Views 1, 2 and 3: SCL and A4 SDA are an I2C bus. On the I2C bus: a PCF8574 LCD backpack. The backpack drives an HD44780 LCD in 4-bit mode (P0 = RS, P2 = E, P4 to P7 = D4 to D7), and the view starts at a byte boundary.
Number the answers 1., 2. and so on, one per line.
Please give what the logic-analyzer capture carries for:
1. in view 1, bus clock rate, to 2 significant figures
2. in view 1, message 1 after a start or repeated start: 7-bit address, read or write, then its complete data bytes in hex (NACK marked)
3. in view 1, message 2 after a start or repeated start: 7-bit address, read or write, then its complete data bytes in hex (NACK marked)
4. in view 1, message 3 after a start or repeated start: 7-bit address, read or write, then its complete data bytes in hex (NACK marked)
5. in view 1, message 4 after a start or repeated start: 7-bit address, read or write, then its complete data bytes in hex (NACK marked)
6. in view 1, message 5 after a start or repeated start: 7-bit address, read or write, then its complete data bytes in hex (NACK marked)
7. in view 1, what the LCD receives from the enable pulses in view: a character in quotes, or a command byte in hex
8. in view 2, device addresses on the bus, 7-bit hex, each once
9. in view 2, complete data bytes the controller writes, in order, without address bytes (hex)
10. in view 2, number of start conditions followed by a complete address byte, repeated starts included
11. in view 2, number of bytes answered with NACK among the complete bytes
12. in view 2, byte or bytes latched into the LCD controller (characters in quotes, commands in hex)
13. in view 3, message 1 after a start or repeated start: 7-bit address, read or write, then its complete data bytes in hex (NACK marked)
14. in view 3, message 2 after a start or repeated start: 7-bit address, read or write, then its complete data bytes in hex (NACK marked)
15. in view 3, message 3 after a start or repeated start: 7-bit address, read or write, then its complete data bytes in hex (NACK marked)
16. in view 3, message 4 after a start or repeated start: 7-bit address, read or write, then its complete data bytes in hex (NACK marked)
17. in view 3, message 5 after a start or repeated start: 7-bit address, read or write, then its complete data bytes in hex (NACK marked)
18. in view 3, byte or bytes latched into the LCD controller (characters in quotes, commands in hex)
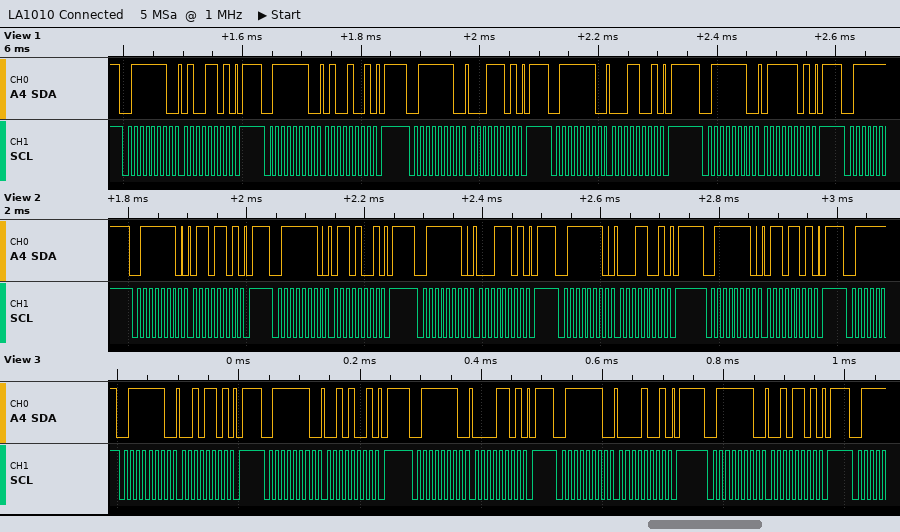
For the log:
1. 100 kHz
2. 0x3F write: 4D
3. 0x3F write: 49
4. 0x3F write: 1D
5. 0x3F write: 19
6. 0x3F write: 7D
7. 'A'
8. 0x3F
9. 6D 69 1D 19 6D
10. 5
11. 0
12. 'a'
13. 0x3F write: 2D
14. 0x3F write: 29
15. 0x3F write: 0D
16. 0x3F write: 09
17. 0x3F write: 2D
18. ' '
